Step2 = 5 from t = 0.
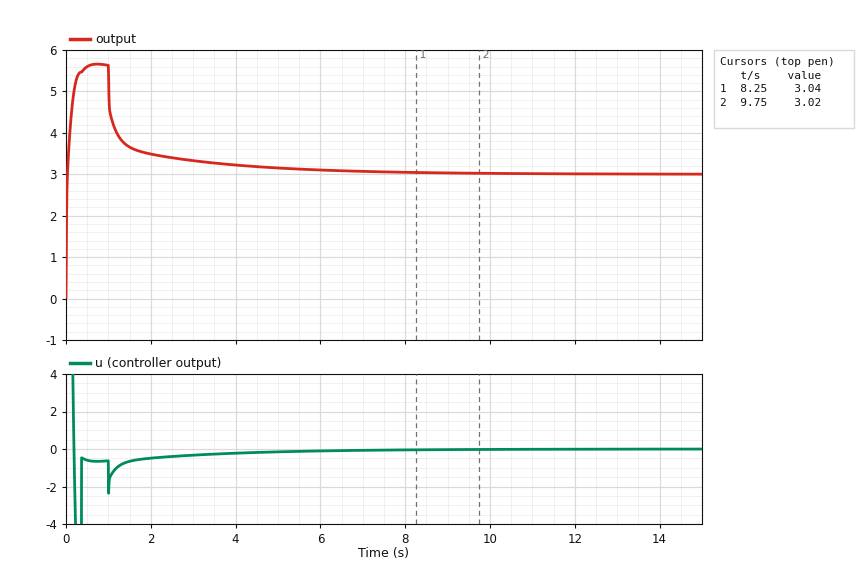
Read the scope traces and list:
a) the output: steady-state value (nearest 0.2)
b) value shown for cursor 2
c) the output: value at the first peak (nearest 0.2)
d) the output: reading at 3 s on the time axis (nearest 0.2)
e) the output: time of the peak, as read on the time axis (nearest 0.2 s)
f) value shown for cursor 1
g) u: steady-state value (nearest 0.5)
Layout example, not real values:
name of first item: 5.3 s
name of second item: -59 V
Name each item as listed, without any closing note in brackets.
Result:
the output: steady-state value: 3.0
value shown for cursor 2: 3.02
the output: value at the first peak: 5.6
the output: reading at 3 s on the time axis: 3.4
the output: time of the peak, as read on the time axis: 0.8 s
value shown for cursor 1: 3.04
u: steady-state value: 0.0
